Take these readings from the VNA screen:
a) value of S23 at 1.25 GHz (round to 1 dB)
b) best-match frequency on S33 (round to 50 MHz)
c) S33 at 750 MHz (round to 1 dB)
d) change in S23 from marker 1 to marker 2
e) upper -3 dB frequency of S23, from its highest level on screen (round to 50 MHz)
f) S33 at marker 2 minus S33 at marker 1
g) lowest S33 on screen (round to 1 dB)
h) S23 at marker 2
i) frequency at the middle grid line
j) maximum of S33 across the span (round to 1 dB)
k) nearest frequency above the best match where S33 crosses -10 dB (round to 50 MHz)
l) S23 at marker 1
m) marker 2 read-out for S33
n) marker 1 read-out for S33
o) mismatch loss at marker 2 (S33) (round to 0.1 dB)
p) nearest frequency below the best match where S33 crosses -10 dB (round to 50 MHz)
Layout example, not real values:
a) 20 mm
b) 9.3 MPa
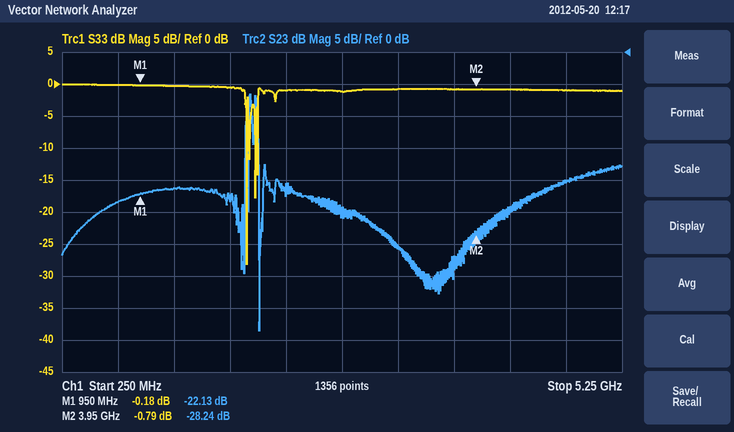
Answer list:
a) -21 dB
b) 1.90 GHz
c) 0 dB
d) -6.11 dB
e) 1.95 GHz
f) -0.61 dB
g) -28 dB
h) -28.24 dB
i) 2.75 GHz
j) 0 dB
k) 1.90 GHz
l) -22.13 dB
m) -0.79 dB
n) -0.18 dB
o) 7.8 dB
p) 1.90 GHz
